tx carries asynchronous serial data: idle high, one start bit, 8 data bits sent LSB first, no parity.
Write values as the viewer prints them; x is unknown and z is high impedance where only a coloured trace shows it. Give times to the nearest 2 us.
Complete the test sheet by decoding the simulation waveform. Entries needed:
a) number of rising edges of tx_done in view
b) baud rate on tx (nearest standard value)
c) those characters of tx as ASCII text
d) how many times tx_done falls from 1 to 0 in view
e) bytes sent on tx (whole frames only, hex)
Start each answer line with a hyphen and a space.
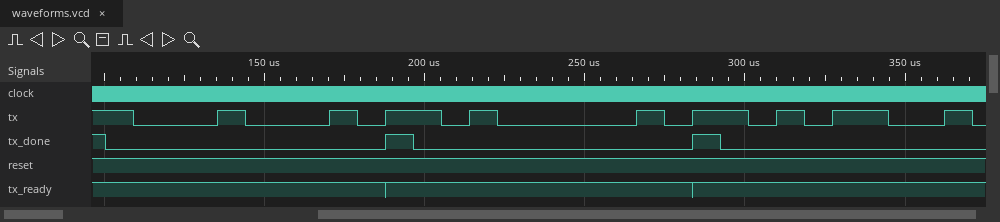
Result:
- 2
- 115200 baud
- "DA"
- 3
- 44, 41
